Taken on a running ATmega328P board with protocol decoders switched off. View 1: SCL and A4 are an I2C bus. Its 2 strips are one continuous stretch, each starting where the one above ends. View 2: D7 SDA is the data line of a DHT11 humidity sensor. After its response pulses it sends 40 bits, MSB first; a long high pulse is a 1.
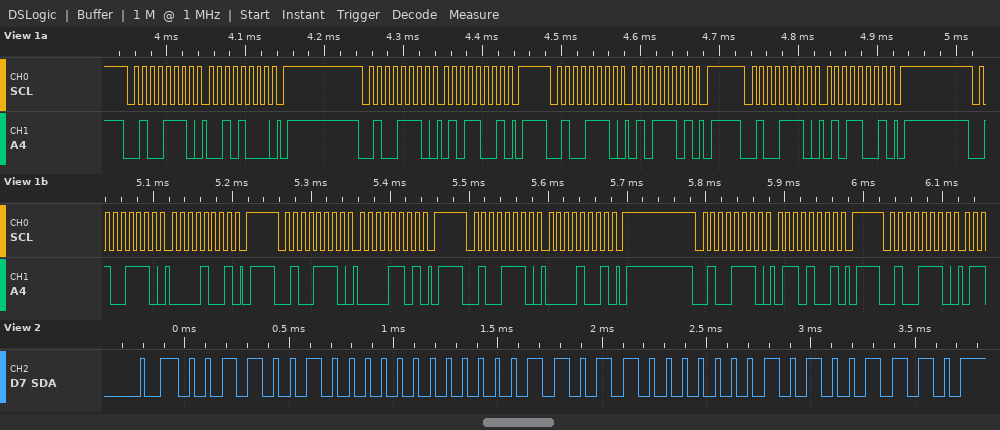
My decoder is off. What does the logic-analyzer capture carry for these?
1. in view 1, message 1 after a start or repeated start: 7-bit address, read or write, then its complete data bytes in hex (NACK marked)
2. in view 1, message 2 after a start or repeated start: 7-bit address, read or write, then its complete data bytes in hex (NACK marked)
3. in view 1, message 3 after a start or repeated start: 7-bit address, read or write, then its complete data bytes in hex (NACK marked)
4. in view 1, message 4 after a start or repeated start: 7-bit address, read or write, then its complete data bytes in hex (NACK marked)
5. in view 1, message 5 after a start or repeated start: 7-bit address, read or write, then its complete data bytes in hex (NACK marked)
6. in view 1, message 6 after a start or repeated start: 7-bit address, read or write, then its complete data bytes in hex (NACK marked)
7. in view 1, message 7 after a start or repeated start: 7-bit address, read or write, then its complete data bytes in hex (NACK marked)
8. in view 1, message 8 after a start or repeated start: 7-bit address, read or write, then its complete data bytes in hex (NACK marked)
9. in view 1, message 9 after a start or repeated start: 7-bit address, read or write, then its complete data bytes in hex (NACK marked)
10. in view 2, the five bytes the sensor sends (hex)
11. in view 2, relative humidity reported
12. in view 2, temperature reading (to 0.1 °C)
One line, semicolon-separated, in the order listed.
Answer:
0x27 write: 28; 0x27 write: 59; 0x27 write: 5D; 0x27 write: 59; 0x27 write: 09; 0x27 write: 0D; 0x27 write: 09; 0x27 write: 69; 0x27 write; 32 00 1B 01 4E; 50 %; 27.1 °C
